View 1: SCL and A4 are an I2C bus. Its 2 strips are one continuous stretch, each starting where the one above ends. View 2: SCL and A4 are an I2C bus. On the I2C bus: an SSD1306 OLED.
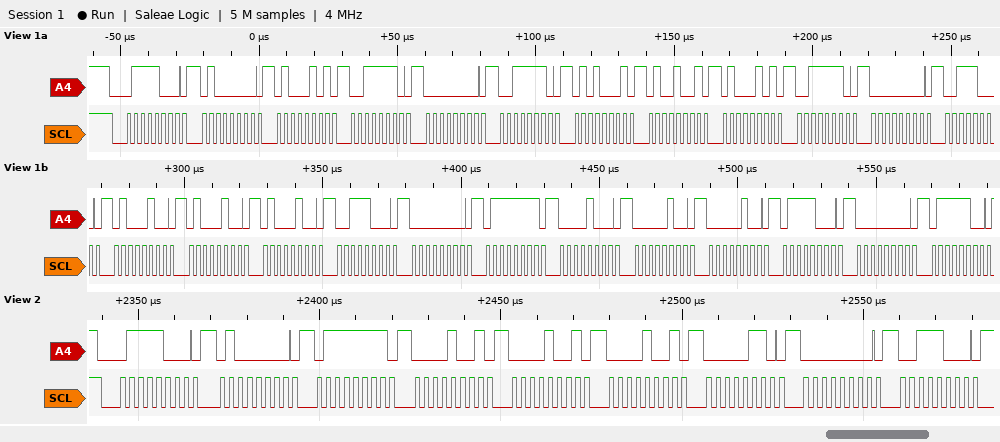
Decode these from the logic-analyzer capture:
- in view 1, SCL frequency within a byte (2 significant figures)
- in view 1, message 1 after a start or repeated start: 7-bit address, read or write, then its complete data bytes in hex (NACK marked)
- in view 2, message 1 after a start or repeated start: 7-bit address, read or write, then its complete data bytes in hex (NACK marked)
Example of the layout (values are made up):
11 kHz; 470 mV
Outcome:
400 kHz; 0x3C write: 40 45 3E 00 3E 51 49 45 3E 00 38 44 44 44 38 00 7F 08 04 04 78 00 7C; 0x3C write: 40 7F 09 09 09 06 00 38
